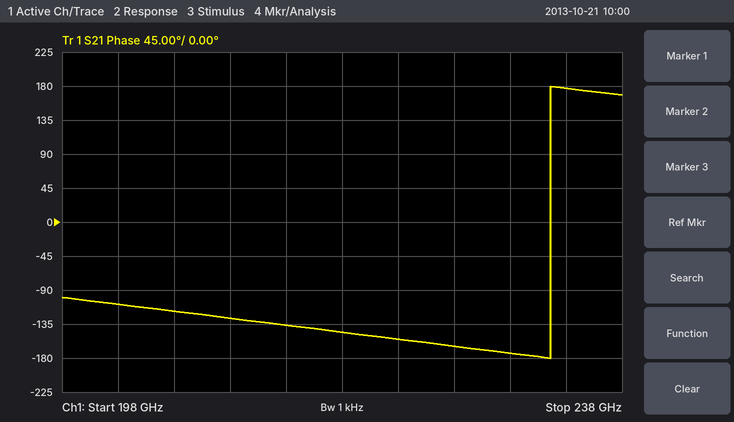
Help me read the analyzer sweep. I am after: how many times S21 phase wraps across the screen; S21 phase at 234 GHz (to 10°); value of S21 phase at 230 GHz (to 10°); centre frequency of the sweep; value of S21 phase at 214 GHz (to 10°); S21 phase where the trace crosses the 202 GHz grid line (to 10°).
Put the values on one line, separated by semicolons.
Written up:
1; 180°; -170°; 218 GHz; -140°; -110°
